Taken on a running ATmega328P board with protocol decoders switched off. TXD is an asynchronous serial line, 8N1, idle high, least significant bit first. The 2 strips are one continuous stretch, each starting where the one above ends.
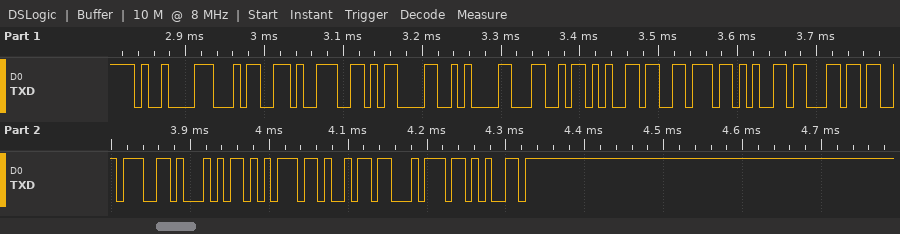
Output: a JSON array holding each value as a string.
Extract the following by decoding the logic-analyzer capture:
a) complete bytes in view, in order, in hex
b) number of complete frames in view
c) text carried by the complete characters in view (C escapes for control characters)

["0x09 0x34 0x39 0x0D 0x0A 0x4C 0x65 0x76 0x65 0x6C 0x3A 0x51 0x75 0x69 0x74 0x65", "16", "\"\\t49\\r\\nLevel:Quite\""]
